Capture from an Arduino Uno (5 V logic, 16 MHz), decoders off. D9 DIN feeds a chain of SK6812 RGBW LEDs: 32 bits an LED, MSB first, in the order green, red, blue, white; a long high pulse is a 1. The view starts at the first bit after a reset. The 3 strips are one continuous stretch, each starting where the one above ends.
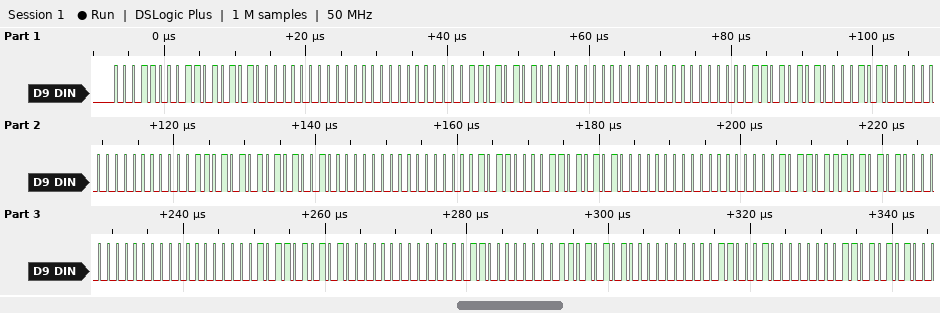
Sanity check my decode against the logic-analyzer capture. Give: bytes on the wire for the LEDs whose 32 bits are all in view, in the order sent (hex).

18 D5 00 00 00 D5 00 00 00 D5 0A 00 00 D5 52 00 00 B0 D5 00 00 2D D5 00 00 02 D5 00 03 00 D5 00
